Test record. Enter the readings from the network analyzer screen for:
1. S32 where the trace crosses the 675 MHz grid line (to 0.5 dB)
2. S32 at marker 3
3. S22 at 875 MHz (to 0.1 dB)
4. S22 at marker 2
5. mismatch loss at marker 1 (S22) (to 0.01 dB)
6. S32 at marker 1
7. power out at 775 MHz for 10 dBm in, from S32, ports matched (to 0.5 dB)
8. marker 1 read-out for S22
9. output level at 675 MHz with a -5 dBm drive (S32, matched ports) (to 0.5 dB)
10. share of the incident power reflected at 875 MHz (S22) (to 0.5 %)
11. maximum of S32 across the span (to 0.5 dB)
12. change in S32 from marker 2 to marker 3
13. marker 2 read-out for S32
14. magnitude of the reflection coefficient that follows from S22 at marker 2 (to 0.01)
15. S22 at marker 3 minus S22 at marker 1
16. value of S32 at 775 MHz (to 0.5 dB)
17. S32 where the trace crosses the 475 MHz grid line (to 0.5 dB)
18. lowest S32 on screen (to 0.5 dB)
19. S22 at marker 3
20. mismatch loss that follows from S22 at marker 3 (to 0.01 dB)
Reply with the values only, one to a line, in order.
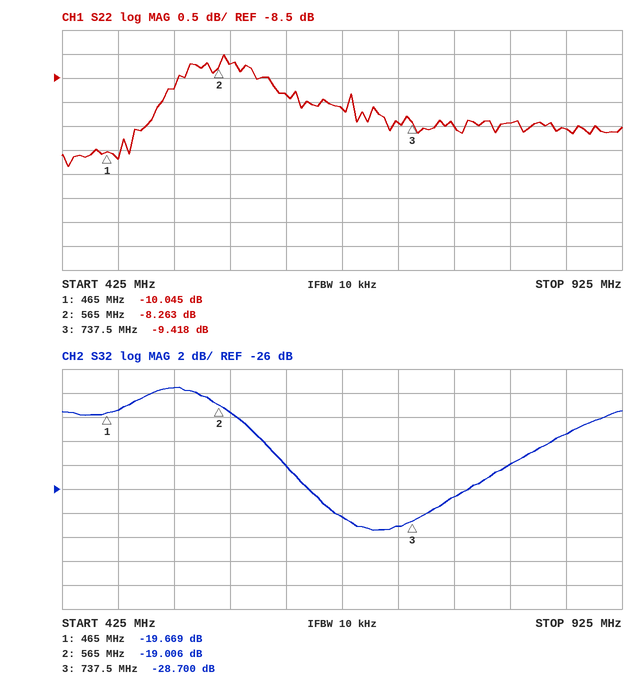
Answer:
-28.5 dB
-28.700 dB
-9.6 dB
-8.263 dB
0.45 dB
-19.669 dB
-16.5 dBm
-10.045 dB
-33.5 dBm
11.0 %
-17.5 dB
-9.694 dB
-19.006 dB
0.39
0.627 dB
-26.5 dB
-19.5 dB
-29.5 dB
-9.418 dB
0.53 dB
